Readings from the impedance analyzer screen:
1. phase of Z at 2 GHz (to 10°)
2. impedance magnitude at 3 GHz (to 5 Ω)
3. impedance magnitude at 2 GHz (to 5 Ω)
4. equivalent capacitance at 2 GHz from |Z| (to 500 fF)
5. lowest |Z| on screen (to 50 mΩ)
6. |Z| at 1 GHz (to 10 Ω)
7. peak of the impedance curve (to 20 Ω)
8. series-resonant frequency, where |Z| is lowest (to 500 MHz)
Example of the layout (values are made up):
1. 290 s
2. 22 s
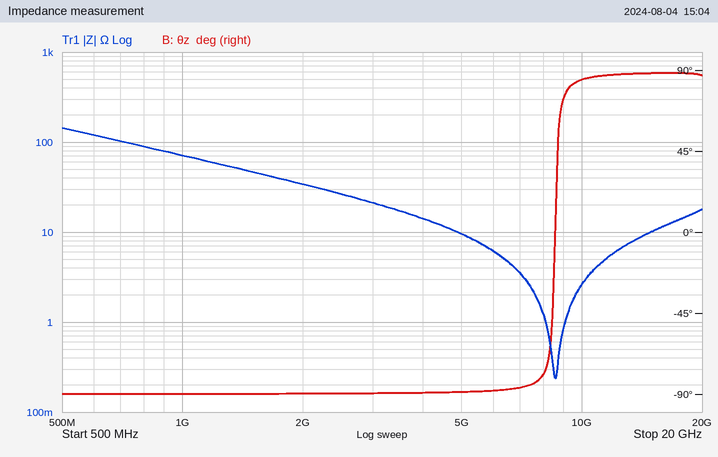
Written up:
1. -90°
2. 20 Ω
3. 35 Ω
4. 2.5 pF
5. 250 mΩ
6. 70 Ω
7. 140 Ω
8. 8.5 GHz
